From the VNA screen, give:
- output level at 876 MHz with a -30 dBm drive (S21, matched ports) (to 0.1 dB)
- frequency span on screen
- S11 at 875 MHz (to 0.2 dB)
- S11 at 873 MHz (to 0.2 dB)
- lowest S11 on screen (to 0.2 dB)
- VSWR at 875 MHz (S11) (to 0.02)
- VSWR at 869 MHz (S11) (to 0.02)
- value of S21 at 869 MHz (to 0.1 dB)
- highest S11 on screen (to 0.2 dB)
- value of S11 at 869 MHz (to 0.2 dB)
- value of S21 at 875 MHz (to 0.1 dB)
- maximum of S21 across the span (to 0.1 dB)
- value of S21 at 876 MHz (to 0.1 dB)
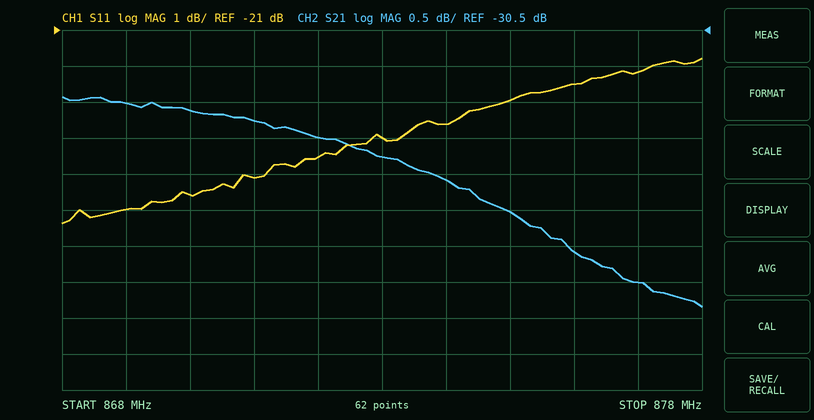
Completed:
-63.6 dBm
10 MHz
-23.0 dB
-24.0 dB
-26.4 dB
1.16
1.10
-31.5 dB
-21.8 dB
-26.0 dB
-33.0 dB
-31.4 dB
-33.6 dB
